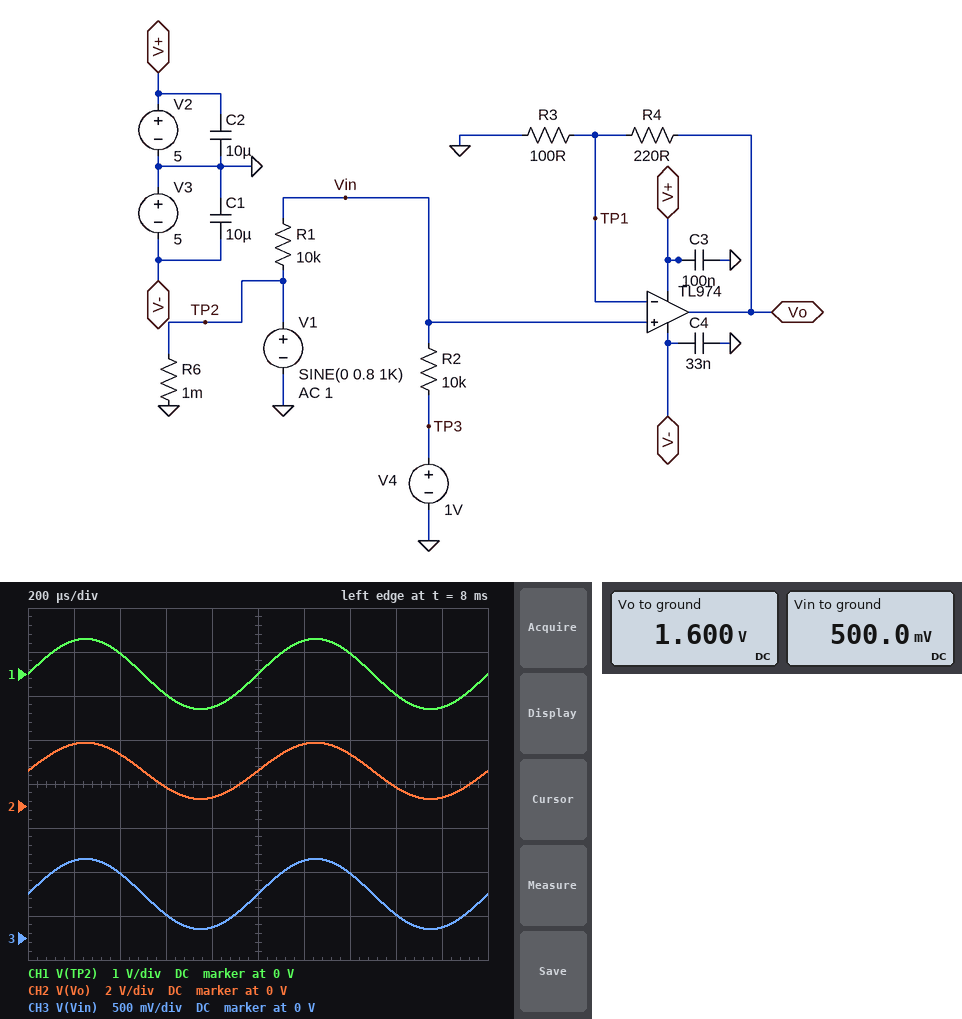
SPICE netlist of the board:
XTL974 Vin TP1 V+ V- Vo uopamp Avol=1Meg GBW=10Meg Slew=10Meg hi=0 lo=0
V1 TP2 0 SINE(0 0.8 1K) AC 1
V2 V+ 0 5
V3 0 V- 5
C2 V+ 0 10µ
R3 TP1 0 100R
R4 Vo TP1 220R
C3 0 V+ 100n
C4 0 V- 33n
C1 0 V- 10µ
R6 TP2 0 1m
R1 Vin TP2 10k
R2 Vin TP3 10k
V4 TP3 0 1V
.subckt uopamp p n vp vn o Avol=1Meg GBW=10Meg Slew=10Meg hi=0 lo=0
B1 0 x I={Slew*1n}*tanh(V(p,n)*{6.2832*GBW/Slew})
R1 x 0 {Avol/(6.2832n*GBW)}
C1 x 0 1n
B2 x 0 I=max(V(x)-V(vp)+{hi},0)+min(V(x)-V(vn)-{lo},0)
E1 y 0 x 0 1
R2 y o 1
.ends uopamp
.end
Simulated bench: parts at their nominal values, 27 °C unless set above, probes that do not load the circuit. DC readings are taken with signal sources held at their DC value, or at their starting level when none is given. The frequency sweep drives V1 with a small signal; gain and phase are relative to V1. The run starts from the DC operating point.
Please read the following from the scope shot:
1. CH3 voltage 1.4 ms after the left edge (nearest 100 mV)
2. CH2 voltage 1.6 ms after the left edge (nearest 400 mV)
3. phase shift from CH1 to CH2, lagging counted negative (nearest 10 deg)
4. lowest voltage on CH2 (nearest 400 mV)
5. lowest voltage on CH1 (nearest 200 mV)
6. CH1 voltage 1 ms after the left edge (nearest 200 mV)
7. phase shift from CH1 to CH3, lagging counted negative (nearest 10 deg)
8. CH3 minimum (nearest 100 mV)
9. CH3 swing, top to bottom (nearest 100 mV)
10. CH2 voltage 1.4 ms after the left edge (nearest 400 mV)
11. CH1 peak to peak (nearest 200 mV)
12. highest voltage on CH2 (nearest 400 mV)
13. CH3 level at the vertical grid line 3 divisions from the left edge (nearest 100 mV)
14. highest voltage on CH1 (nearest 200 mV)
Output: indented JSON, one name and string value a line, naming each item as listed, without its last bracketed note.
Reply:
{
  "CH3 voltage 1.4 ms after the left edge": "700 mV",
  "CH2 voltage 1.6 ms after the left edge": "800 mV",
  "phase shift from CH1 to CH2, lagging counted negative": "0 deg",
  "lowest voltage on CH2": "400 mV",
  "lowest voltage on CH1": "-800 mV",
  "CH1 voltage 1 ms after the left edge": "0 V",
  "phase shift from CH1 to CH3, lagging counted negative": "0 deg",
  "CH3 minimum": "100 mV",
  "CH3 swing, top to bottom": "800 mV",
  "CH2 voltage 1.4 ms after the left edge": "2.4 V",
  "CH1 peak to peak": "1.6 V",
  "highest voltage on CH2": "2.8 V",
  "CH3 level at the vertical grid line 3 divisions from the left edge": "300 mV",
  "highest voltage on CH1": "800 mV"
}
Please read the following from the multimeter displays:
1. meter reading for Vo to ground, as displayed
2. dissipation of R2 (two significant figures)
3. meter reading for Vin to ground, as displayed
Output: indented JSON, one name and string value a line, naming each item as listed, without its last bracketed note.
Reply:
{
  "meter reading for Vo to ground, as displayed": "1.600 V",
  "dissipation of R2": "25 µW",
  "meter reading for Vin to ground, as displayed": "500.0 mV"
}
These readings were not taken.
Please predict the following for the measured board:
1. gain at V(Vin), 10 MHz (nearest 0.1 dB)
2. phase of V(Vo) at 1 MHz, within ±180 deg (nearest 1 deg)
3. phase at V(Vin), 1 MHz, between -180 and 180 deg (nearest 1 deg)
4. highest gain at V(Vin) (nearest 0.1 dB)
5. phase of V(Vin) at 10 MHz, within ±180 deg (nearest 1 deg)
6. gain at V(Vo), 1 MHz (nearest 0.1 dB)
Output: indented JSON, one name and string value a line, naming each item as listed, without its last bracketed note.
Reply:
{
  "gain at V(Vin), 10 MHz": "-6.0 dB",
  "phase of V(Vo) at 1 MHz, within ±180 deg": "-18 deg",
  "phase at V(Vin), 1 MHz, between -180 and 180 deg": "0 deg",
  "highest gain at V(Vin)": "-6.0 dB",
  "phase of V(Vin) at 10 MHz, within ±180 deg": "0 deg",
  "gain at V(Vo), 1 MHz": "3.7 dB"
}
